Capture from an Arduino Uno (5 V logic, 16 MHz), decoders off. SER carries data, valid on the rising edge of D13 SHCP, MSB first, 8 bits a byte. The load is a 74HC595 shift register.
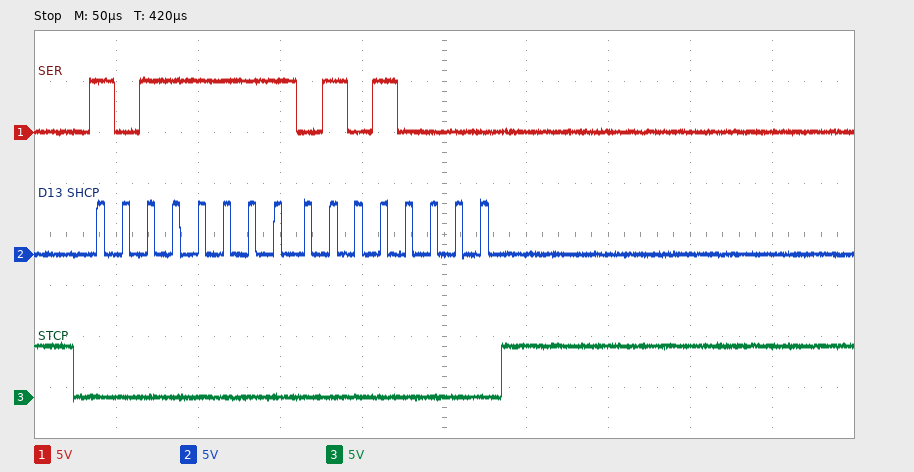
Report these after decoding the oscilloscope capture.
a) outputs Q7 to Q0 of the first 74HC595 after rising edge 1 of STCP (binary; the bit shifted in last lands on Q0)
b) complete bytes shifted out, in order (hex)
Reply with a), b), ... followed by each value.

a) 01010000
b) 0xBF 0x50
